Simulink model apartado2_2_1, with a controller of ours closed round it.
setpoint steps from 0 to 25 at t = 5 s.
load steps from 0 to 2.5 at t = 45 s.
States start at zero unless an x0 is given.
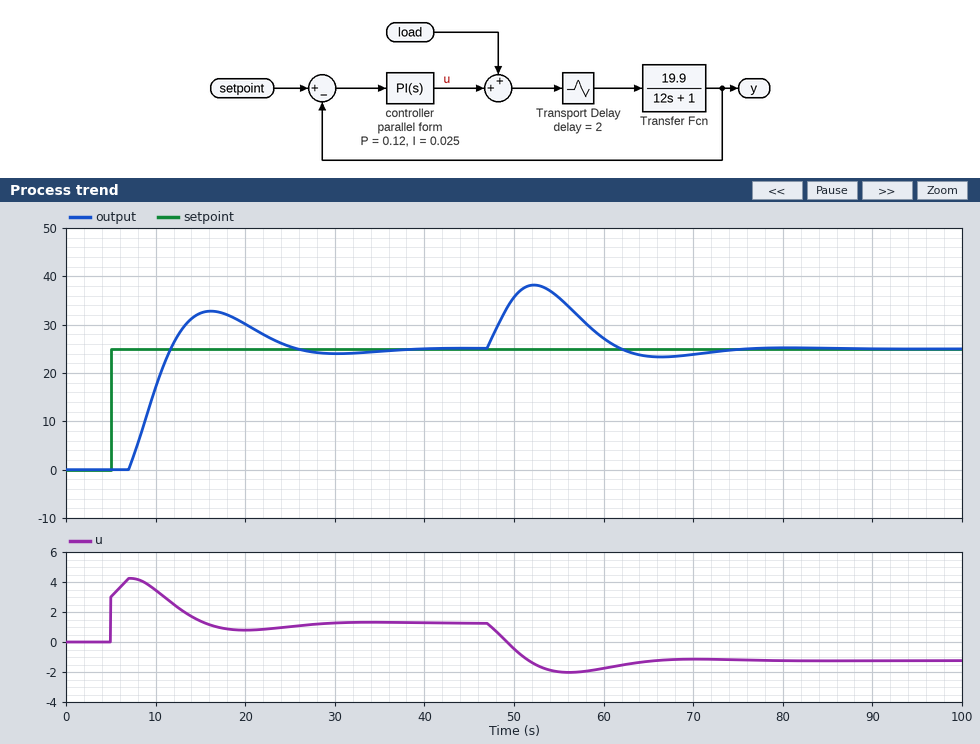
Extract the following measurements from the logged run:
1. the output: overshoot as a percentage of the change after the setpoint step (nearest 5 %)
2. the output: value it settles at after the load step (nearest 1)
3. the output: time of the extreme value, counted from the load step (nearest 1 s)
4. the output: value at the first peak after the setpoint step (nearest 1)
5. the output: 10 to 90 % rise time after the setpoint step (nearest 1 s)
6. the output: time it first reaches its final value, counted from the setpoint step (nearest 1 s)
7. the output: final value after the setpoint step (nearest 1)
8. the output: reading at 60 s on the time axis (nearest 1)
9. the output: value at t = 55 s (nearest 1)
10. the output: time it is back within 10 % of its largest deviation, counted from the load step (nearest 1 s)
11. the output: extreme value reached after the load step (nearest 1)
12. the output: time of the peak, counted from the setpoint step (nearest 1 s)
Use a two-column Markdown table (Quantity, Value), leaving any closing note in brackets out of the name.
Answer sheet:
| Quantity | Value |
|---|---|
| the output: overshoot as a percentage of the change after the setpoint step | 30 % |
| the output: value it settles at after the load step | 25 |
| the output: time of the extreme value, counted from the load step | 7 s |
| the output: value at the first peak after the setpoint step | 33 |
| the output: 10 to 90 % rise time after the setpoint step | 4 s |
| the output: time it first reaches its final value, counted from the setpoint step | 7 s |
| the output: final value after the setpoint step | 25 |
| the output: reading at 60 s on the time axis | 27 |
| the output: value at t = 55 s | 36 |
| the output: time it is back within 10 % of its largest deviation, counted from the load step | 24 s |
| the output: extreme value reached after the load step | 38 |
| the output: time of the peak, counted from the setpoint step | 11 s |
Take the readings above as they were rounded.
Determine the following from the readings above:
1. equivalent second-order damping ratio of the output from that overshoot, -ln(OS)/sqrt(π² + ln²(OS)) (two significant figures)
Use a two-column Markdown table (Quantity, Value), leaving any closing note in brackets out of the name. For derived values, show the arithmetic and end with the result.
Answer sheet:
| Quantity | Value |
|---|---|
| equivalent second-order damping ratio of the output from that overshoot, -ln(OS)/sqrt(π² + ln²(OS)) | ln(0.3) = -1.204; 1.204 / sqrt(9.870 + 1.450) = 0.36 |
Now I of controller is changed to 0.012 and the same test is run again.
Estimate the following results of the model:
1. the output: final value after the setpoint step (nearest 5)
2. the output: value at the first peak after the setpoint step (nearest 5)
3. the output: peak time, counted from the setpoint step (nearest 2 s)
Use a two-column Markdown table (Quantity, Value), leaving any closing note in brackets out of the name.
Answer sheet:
| Quantity | Value |
|---|---|
| the output: final value after the setpoint step | 25 |
| the output: value at the first peak after the setpoint step | 25 |
| the output: peak time, counted from the setpoint step | 14 s |
